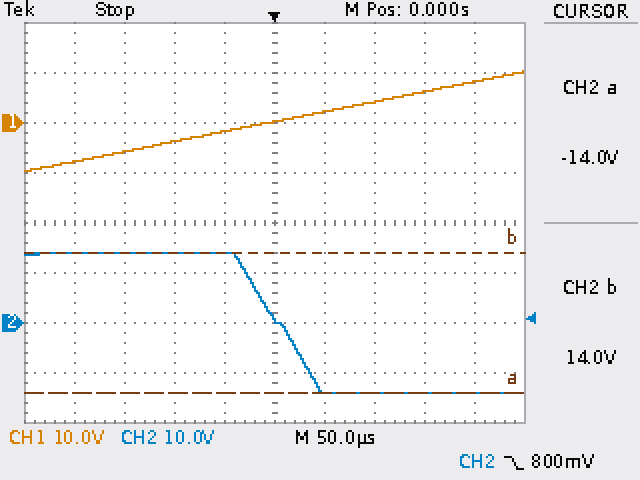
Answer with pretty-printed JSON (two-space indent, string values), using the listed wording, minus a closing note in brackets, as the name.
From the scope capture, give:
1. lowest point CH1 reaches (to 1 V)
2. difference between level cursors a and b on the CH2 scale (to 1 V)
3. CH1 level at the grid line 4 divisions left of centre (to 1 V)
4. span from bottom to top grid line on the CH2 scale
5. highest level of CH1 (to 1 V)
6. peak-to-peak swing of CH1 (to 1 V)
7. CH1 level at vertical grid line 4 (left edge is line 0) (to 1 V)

{
  "lowest point CH1 reaches": "-10 V",
  "difference between level cursors a and b on the CH2 scale": "28 V",
  "CH1 level at the grid line 4 divisions left of centre": "-8 V",
  "span from bottom to top grid line on the CH2 scale": "80 V",
  "highest level of CH1": "10 V",
  "peak-to-peak swing of CH1": "20 V",
  "CH1 level at vertical grid line 4 (left edge is line 0)": "-2 V"
}
